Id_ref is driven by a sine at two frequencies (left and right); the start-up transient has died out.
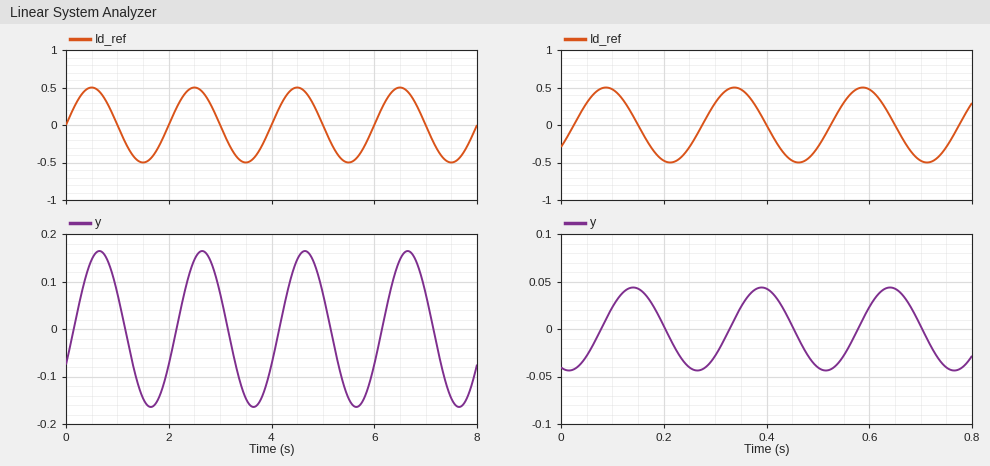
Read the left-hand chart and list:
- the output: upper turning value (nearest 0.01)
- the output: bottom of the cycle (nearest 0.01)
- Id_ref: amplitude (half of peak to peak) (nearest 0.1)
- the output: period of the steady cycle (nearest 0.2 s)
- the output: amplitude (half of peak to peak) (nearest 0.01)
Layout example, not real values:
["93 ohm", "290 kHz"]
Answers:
["0.16", "-0.16", "0.5", "2.0 s", "0.16"]
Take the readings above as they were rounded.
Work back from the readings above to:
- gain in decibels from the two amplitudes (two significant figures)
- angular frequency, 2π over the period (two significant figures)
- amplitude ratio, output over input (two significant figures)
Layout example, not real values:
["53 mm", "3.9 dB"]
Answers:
["-9.9 dB", "3.1 rad/s", "0.32"]
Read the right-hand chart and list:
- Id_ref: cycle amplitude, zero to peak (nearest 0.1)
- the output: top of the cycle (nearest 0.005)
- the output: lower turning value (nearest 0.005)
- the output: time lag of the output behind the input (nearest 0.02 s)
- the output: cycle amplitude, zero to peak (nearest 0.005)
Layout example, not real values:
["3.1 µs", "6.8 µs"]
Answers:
["0.5", "0.045", "-0.045", "0.06 s", "0.045"]
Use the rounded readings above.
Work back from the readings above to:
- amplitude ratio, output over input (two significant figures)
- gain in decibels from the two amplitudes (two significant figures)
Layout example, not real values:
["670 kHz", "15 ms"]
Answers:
["0.090", "-21 dB"]
